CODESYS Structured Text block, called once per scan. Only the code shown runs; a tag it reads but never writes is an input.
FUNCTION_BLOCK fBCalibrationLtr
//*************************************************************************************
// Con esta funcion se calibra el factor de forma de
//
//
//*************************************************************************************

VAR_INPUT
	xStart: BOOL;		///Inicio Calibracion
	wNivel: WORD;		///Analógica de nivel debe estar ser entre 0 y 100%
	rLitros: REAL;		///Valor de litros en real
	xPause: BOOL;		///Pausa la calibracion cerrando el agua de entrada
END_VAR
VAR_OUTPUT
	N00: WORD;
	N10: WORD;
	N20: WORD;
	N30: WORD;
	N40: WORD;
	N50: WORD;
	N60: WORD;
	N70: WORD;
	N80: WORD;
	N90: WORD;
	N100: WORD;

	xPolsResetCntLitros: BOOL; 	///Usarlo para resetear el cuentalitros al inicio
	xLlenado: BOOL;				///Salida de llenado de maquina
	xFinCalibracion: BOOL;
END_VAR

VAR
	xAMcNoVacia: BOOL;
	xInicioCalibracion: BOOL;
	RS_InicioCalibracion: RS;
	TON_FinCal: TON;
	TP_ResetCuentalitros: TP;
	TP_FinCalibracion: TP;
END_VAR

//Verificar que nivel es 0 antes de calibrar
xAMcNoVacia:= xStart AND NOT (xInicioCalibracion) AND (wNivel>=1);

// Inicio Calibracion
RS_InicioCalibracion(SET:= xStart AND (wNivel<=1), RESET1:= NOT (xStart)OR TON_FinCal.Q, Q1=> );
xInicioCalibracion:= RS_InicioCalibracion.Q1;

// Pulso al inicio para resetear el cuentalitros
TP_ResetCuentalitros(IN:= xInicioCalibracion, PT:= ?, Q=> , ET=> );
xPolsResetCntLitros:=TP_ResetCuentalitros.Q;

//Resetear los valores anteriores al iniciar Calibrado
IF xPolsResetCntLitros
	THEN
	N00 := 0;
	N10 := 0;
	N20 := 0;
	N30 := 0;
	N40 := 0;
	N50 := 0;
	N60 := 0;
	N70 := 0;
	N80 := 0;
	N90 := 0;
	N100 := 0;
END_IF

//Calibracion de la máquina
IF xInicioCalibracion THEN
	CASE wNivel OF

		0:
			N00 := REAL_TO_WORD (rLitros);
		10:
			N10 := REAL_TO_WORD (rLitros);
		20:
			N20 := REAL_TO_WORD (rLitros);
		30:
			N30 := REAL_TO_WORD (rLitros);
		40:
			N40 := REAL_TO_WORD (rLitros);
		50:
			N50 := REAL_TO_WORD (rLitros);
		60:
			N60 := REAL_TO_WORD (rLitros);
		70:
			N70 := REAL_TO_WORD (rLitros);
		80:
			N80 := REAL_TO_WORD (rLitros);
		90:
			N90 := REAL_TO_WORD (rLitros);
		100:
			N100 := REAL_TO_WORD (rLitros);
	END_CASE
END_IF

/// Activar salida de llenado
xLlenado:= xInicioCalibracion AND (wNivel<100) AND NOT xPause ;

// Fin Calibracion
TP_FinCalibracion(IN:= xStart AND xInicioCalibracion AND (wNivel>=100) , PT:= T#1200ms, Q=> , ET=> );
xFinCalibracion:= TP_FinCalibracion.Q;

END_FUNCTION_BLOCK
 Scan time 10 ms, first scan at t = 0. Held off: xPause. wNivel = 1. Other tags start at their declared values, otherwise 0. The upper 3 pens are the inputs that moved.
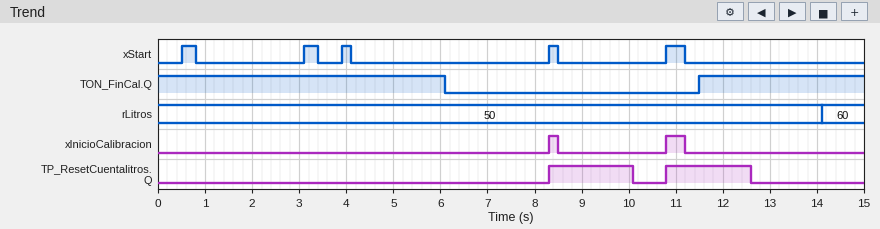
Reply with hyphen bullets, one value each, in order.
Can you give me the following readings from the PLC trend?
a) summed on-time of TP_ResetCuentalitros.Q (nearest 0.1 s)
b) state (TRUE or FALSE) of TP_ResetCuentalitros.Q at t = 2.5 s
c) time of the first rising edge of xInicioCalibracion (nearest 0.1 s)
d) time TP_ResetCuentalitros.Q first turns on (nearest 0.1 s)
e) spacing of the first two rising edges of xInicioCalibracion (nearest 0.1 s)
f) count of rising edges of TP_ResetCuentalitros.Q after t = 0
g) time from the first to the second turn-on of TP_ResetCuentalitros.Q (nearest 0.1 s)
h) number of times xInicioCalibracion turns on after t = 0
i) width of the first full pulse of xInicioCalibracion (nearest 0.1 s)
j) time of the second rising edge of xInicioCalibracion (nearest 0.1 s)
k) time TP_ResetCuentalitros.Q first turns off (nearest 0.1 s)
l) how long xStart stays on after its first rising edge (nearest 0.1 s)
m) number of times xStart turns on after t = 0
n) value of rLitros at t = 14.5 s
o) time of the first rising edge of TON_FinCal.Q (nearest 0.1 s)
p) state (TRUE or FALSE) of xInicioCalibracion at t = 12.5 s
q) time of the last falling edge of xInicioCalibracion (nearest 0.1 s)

- 3.6 s
- FALSE
- 8.3 s
- 8.3 s
- 2.5 s
- 2
- 2.5 s
- 2
- 0.2 s
- 10.8 s
- 10.1 s
- 0.3 s
- 5
- 60
- 11.5 s
- FALSE
- 11.2 s
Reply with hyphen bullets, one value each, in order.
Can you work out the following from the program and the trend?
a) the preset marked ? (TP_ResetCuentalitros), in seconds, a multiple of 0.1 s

- 1.8 s
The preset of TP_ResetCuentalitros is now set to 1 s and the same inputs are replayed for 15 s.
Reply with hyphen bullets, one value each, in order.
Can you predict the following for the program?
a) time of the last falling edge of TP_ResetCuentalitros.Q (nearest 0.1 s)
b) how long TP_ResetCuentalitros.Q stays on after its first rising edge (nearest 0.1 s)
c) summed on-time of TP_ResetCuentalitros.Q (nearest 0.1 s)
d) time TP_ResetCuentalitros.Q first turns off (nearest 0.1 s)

- 11.8 s
- 1.0 s
- 2.0 s
- 9.3 s
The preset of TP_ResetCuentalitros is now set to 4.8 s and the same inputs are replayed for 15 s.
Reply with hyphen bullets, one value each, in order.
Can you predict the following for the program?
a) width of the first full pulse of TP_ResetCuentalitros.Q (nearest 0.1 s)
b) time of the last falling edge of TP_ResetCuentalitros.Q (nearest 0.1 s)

- 4.8 s
- 13.1 s
